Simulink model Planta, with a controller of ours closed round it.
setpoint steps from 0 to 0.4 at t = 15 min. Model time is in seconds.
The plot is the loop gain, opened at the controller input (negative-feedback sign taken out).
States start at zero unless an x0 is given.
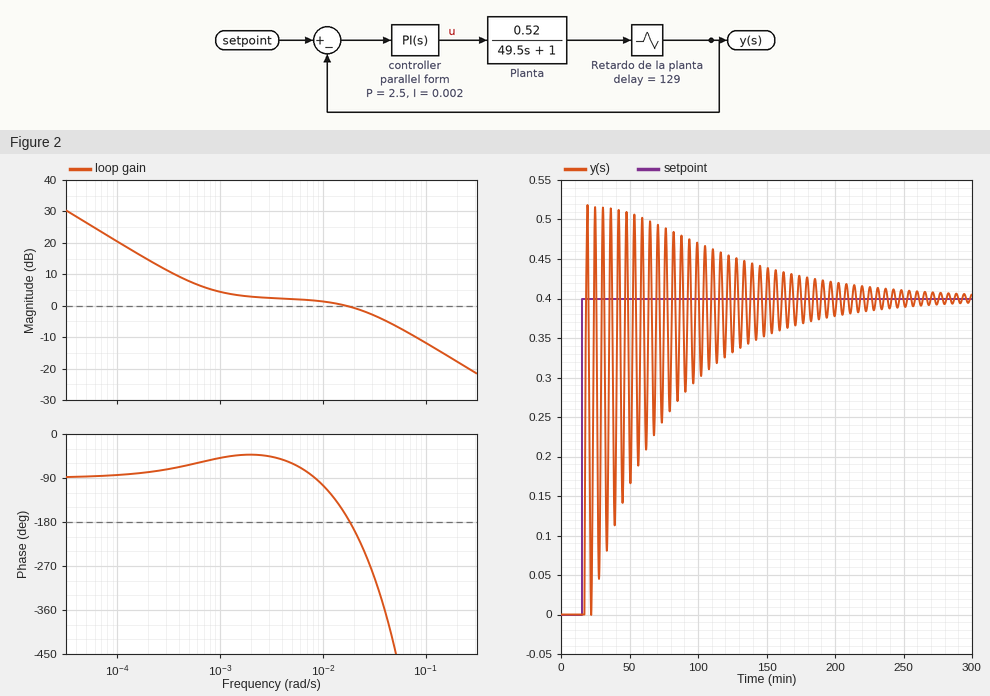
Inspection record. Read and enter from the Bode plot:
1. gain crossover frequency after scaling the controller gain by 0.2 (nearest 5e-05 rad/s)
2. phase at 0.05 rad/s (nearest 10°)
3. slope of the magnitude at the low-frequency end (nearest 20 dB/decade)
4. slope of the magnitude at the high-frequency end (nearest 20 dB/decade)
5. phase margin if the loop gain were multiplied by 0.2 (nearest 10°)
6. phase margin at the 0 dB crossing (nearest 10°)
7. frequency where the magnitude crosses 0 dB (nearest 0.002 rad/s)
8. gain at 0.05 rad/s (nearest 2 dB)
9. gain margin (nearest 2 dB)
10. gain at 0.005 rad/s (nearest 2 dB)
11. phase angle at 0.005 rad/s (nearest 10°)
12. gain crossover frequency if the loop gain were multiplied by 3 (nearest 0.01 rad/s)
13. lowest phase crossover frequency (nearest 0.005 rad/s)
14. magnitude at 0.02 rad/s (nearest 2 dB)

0.00020 rad/s
-440°
-20 dB/decade
-20 dB/decade
100°
10°
0.016 rad/s
-6 dB
0 dB
2 dB
-60°
0.08 rad/s
0.020 rad/s
0 dB
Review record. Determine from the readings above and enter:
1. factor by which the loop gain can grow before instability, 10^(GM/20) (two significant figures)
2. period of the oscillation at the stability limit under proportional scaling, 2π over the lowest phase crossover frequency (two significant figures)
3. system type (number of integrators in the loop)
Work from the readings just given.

1.0
310 s
1
